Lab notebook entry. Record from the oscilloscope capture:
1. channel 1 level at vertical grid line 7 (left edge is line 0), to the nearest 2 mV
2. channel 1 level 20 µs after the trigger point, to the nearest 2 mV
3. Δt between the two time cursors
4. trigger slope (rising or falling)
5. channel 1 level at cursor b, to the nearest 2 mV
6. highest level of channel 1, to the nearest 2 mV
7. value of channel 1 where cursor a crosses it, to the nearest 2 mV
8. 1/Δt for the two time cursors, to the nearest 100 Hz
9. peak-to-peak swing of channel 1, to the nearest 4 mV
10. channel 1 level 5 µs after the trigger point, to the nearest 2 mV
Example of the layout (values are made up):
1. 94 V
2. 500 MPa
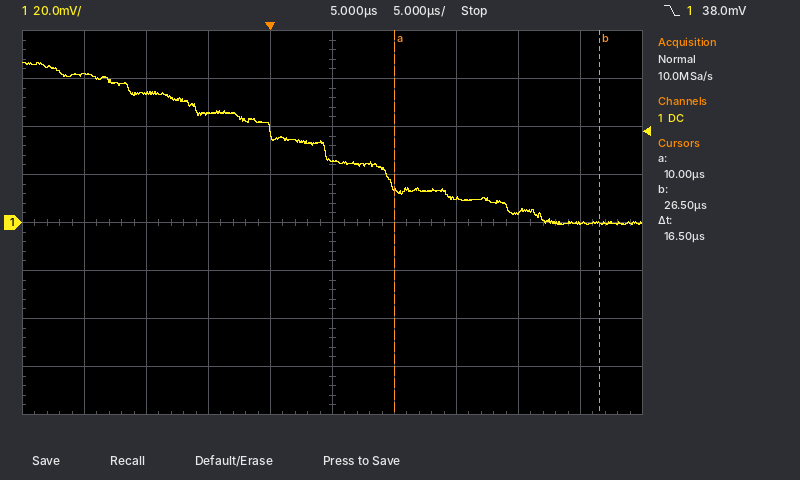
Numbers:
1. 10 mV
2. 4 mV
3. 16.5 µs
4. falling
5. 0 mV
6. 66 mV
7. 14 mV
8. 60.6 kHz
9. 68 mV
10. 26 mV
